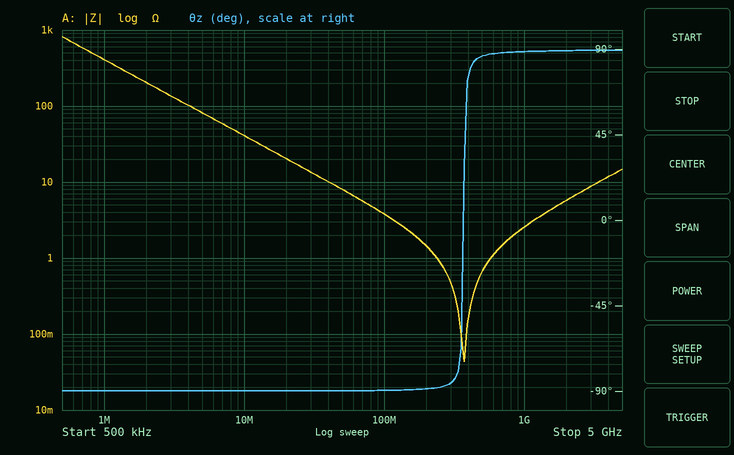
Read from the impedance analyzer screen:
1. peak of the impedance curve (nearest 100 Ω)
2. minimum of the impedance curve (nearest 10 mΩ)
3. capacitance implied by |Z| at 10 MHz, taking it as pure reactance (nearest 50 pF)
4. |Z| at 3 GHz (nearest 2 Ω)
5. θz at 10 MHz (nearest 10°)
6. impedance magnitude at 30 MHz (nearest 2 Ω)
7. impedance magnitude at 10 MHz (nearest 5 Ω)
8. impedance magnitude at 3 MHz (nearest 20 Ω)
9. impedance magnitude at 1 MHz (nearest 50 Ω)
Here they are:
800 Ω
40 mΩ
400 pF
8 Ω
-90°
14 Ω
40 Ω
140 Ω
400 Ω
